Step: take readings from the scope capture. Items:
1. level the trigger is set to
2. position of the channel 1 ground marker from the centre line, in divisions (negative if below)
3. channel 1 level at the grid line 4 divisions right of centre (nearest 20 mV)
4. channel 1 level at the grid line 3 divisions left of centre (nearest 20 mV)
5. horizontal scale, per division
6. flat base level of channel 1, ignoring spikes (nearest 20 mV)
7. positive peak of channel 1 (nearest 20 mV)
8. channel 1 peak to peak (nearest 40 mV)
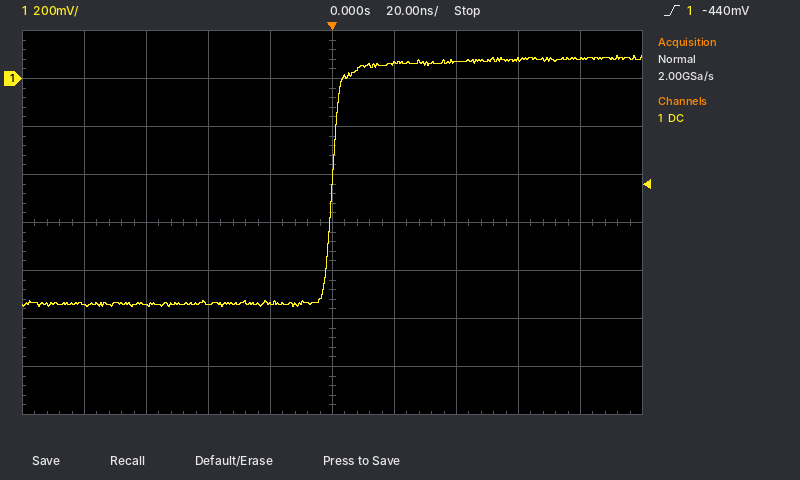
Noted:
-440 mV
+3.0 div
80 mV
-940 mV
20 ns
-940 mV
100 mV
1.04 V
